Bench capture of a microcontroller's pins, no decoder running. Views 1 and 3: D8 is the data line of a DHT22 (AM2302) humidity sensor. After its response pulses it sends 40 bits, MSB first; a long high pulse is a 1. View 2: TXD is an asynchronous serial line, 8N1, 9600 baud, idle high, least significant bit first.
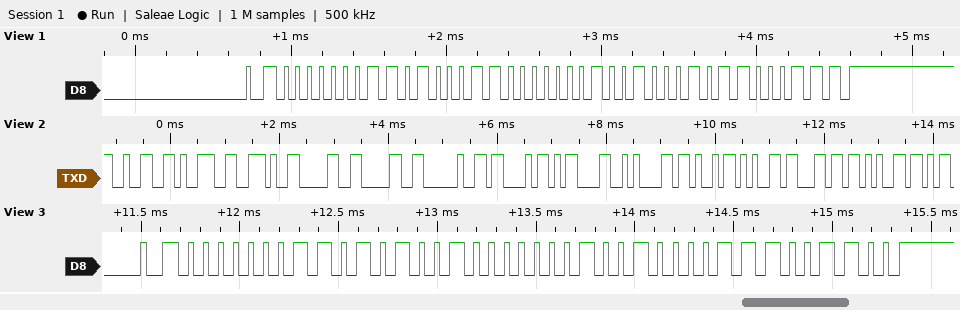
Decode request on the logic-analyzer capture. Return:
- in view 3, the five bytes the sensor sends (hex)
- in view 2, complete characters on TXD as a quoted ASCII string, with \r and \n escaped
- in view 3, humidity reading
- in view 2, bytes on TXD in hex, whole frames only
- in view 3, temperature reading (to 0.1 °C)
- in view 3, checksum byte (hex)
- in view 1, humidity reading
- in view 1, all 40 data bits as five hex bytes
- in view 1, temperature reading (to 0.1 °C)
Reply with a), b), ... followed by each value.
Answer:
a) 01 A9 01 21 CC
b) "29.00 C\r\nKele"
c) 42.5 %
d) 32 39 2E 30 30 20 43 0D 0A 4B 65 6C 65
e) 28.9 °C
f) 0xCC
g) 41.9 %
h) 01 A3 01 22 C7
i) 29.0 °C
